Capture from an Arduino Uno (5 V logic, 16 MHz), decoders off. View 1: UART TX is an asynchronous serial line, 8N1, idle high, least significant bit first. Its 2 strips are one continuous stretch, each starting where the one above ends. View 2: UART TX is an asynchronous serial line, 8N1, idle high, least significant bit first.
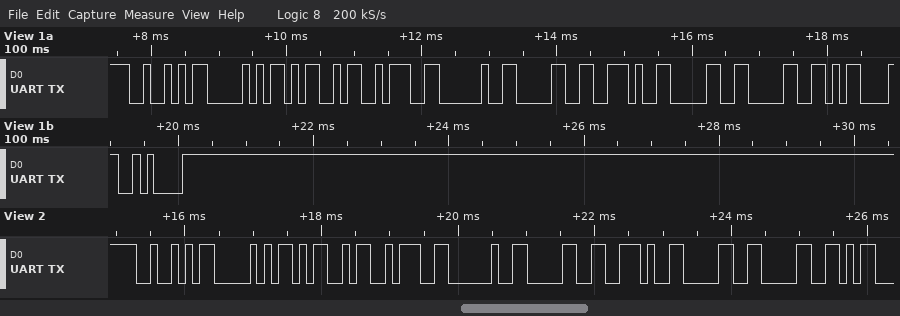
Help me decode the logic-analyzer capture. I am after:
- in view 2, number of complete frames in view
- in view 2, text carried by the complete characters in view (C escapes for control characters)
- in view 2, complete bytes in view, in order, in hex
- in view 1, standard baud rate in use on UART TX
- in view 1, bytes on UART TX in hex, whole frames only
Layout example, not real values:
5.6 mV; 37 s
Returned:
9; "RPM: 0.00"; 52 50 4D 3A 20 30 2E 30 30; 9600 baud; 0x52 0x50 0x4D 0x3A 0x20 0x30 0x2E 0x30 0x30 0x0D 0x0A
